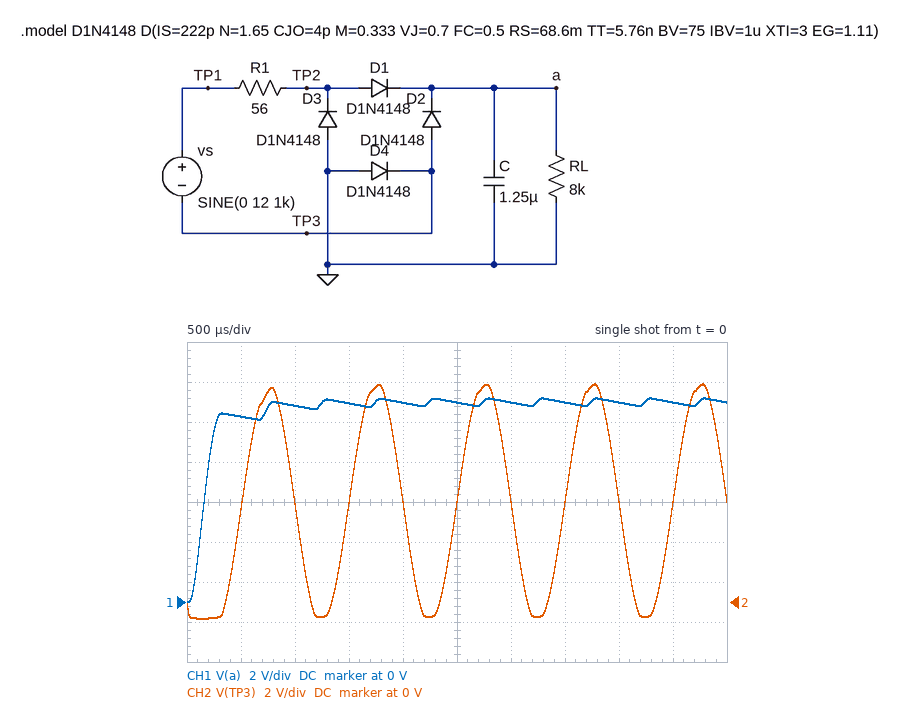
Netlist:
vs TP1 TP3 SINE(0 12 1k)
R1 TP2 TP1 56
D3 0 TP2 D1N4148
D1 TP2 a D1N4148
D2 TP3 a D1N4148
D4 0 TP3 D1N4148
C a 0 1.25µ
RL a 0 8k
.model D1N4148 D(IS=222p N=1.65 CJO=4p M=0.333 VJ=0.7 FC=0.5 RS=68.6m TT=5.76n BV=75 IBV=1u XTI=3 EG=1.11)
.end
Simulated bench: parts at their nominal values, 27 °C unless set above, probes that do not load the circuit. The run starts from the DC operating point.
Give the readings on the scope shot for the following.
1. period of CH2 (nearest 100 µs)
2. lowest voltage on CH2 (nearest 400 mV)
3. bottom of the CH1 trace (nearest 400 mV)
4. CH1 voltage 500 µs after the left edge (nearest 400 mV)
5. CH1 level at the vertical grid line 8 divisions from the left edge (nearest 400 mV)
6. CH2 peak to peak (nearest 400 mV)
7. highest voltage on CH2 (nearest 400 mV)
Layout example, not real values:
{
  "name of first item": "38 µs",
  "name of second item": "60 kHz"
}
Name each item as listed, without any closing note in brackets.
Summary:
{
  "period of CH2": "1.0 ms",
  "lowest voltage on CH2": "-800 mV",
  "bottom of the CH1 trace": "0 V",
  "CH1 voltage 500 µs after the left edge": "9.2 V",
  "CH1 level at the vertical grid line 8 divisions from the left edge": "10.0 V",
  "CH2 peak to peak": "11.6 V",
  "highest voltage on CH2": "10.8 V"
}
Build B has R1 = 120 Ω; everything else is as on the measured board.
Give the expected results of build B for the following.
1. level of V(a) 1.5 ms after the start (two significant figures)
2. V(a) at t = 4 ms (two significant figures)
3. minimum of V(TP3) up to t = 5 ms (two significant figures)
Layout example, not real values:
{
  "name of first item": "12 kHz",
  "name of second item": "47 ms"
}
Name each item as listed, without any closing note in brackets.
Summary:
{
  "level of V(a) 1.5 ms after the start": "9.4 V",
  "V(a) at t = 4 ms": "9.7 V",
  "minimum of V(TP3) up to t = 5 ms": "-820 mV"
}
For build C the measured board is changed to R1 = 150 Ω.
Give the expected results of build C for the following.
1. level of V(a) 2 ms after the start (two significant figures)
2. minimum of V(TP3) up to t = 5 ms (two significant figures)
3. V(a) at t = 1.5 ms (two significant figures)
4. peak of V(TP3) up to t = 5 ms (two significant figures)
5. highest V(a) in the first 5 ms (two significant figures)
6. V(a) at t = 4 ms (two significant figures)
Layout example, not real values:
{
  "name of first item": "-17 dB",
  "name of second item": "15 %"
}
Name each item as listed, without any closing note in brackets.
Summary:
{
  "level of V(a) 2 ms after the start": "9.3 V",
  "minimum of V(TP3) up to t = 5 ms": "-810 mV",
  "V(a) at t = 1.5 ms": "9.1 V",
  "peak of V(TP3) up to t = 5 ms": "10 V",
  "highest V(a) in the first 5 ms": "9.7 V",
  "V(a) at t = 4 ms": "9.5 V"
}
